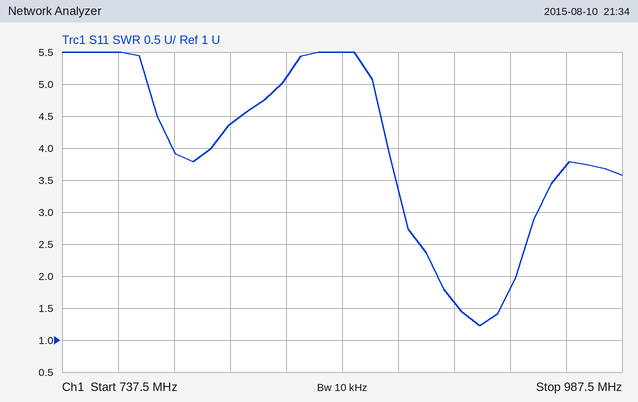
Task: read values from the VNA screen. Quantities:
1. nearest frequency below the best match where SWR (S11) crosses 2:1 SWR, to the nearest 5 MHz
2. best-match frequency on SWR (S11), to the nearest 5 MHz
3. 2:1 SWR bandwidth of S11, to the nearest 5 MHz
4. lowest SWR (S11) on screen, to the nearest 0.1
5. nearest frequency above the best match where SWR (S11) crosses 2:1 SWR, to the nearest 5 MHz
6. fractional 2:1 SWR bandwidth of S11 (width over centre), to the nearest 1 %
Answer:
905 MHz
925 MHz
35 MHz
1.2
940 MHz
4 %
